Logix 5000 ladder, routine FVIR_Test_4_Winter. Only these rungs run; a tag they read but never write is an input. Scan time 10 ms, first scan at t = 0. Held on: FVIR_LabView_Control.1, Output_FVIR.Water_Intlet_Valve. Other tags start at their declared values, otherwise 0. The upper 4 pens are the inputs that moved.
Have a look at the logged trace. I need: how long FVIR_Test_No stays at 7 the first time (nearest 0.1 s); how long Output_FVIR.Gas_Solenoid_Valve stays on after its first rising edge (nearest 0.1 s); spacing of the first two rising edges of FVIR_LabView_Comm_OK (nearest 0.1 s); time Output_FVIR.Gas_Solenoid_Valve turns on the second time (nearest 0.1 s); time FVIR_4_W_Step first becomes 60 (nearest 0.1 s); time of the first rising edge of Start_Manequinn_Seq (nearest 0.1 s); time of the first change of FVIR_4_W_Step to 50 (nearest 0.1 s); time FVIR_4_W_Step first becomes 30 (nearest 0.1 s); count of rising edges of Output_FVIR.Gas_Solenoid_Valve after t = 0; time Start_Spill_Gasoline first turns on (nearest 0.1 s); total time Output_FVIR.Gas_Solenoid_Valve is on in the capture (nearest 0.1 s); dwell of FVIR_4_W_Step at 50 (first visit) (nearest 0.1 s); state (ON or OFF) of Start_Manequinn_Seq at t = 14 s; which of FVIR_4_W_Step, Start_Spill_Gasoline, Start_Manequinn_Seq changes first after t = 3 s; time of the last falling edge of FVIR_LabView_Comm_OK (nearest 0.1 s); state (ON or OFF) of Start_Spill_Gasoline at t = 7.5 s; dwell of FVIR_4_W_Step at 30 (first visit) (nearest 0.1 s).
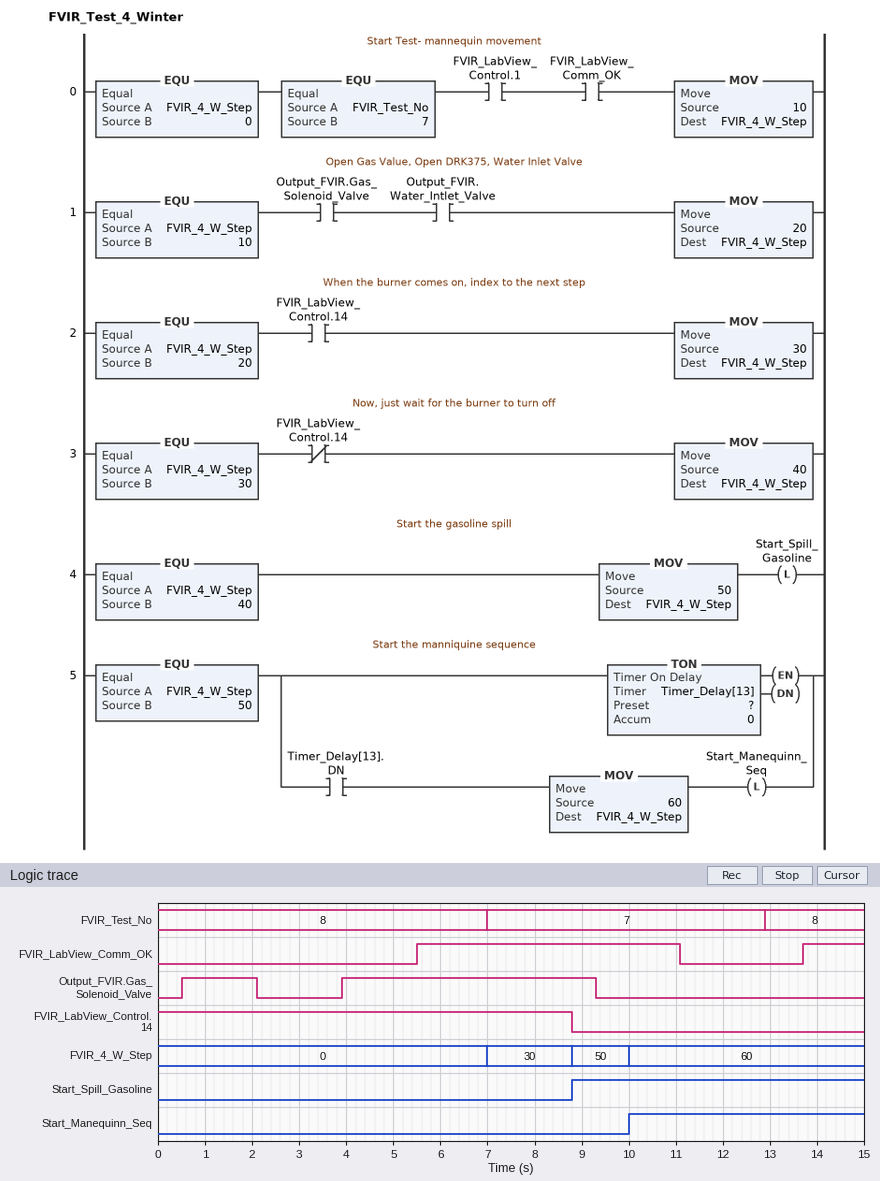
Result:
5.9 s
1.6 s
8.2 s
3.9 s
10.0 s
10.0 s
8.8 s
7.0 s
2
8.8 s
7.0 s
1.2 s
ON
FVIR_4_W_Step
11.1 s
OFF
1.8 s
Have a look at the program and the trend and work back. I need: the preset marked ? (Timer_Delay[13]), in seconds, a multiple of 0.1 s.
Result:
1.2 s
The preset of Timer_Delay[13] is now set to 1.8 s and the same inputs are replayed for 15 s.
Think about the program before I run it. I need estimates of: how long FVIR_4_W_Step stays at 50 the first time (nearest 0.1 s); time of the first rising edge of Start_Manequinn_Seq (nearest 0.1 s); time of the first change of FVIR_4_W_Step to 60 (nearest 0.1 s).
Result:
1.8 s
10.6 s
10.6 s
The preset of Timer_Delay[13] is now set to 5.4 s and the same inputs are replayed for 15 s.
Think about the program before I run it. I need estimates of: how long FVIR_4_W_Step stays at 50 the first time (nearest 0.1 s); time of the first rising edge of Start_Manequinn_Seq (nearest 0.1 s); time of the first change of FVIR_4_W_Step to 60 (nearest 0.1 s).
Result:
5.4 s
14.2 s
14.2 s
